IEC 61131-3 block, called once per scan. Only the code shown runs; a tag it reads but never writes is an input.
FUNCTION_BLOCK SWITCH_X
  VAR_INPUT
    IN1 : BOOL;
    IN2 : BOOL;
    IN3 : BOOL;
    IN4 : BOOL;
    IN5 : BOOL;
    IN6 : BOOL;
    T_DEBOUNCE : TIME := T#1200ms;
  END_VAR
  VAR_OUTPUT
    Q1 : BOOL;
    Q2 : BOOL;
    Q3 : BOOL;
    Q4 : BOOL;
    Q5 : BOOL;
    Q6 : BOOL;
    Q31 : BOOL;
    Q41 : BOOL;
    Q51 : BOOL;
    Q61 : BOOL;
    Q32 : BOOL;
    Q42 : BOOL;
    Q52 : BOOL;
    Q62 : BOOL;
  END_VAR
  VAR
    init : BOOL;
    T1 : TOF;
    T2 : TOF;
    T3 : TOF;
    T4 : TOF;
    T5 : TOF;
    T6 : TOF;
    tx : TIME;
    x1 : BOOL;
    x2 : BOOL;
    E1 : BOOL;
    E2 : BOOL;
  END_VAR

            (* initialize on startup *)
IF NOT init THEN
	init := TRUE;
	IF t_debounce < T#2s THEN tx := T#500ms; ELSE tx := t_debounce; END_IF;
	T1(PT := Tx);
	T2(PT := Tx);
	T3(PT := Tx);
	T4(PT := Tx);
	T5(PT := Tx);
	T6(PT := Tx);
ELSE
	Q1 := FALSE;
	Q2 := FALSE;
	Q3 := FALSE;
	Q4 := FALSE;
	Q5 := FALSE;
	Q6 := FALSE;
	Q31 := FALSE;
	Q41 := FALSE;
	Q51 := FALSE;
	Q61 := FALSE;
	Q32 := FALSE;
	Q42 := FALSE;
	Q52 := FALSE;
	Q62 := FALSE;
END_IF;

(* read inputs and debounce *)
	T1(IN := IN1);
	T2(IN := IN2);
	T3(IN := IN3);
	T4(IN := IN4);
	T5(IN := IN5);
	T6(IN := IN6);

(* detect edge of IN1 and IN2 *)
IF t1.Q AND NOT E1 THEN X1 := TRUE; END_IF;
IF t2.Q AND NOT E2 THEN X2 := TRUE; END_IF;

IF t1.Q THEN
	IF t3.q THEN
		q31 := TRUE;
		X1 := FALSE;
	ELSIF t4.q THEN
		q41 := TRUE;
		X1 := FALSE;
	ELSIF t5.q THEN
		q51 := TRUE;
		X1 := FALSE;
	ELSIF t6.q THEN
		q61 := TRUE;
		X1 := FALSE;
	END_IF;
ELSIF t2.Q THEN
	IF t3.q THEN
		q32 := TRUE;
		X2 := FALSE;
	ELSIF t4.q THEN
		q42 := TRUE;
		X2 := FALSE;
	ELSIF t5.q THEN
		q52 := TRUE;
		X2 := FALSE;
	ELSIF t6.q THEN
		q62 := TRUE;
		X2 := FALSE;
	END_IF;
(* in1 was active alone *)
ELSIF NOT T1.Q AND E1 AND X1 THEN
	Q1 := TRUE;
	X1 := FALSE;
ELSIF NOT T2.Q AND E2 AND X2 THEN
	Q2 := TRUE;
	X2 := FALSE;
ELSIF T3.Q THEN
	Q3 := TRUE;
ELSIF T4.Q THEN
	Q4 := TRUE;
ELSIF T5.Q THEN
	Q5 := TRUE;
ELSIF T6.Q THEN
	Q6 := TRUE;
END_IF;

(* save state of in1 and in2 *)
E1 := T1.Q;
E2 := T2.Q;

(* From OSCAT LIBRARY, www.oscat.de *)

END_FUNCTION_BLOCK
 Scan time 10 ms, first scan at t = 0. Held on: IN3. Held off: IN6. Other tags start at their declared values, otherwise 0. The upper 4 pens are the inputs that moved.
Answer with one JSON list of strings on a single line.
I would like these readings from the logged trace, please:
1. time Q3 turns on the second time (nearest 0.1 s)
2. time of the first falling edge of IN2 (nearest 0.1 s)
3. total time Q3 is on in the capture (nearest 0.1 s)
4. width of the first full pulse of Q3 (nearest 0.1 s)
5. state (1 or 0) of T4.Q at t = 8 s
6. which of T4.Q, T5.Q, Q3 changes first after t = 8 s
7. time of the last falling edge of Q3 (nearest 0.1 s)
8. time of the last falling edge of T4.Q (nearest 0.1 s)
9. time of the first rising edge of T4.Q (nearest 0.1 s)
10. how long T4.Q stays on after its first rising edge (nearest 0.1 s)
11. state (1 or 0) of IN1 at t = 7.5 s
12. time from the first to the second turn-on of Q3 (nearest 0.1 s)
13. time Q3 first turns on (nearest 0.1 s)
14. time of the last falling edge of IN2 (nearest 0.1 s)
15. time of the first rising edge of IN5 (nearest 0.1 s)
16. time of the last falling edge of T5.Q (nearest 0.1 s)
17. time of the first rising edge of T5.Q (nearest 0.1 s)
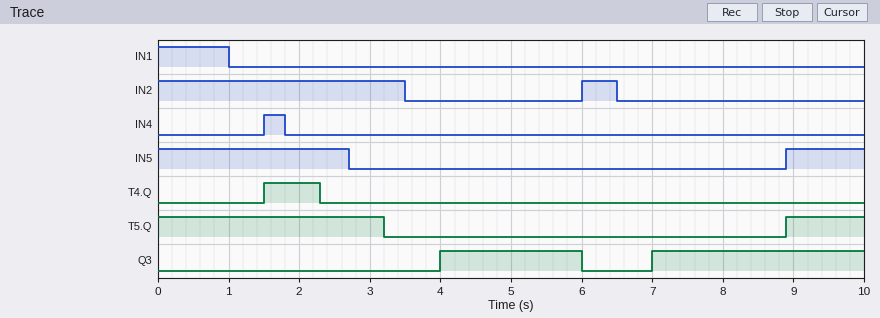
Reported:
["7.0 s", "3.5 s", "5.0 s", "2.0 s", "0", "T5.Q", "6.0 s", "2.3 s", "1.5 s", "0.8 s", "0", "3.0 s", "4.0 s", "6.5 s", "8.9 s", "3.2 s", "8.9 s"]
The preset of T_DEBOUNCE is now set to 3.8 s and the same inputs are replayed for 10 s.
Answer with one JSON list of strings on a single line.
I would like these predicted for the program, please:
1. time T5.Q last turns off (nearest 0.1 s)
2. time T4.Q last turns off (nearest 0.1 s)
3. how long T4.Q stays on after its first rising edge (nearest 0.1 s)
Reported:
["6.5 s", "5.6 s", "4.1 s"]
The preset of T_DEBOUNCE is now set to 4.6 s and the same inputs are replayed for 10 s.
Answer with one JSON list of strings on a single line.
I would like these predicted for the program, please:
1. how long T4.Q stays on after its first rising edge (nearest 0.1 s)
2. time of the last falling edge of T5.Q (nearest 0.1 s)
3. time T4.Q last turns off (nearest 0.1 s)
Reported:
["4.9 s", "7.3 s", "6.4 s"]
